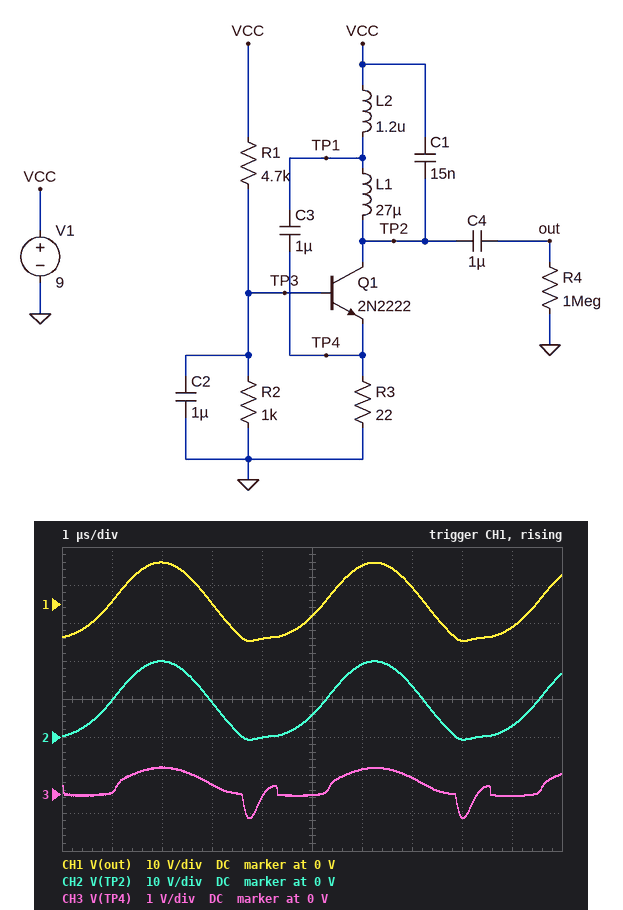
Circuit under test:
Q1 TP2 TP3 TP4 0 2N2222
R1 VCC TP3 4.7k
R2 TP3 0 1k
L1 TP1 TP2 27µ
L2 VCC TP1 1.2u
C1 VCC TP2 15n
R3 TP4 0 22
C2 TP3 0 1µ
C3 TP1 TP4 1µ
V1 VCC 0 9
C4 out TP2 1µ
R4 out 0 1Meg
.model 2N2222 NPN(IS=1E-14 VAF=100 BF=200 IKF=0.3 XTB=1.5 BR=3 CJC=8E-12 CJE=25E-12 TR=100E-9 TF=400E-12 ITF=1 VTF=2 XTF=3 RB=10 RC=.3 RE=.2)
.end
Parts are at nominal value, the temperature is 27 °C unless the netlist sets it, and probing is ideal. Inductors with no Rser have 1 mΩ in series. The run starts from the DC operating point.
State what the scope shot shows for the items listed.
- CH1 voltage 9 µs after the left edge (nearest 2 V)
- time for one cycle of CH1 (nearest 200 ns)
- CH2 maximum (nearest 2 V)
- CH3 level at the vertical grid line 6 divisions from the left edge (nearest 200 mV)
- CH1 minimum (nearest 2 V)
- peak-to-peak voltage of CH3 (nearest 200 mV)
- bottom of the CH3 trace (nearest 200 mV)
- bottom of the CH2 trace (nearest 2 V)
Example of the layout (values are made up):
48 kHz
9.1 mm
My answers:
-6 V
4.2 µs
20 V
600 mV
-10 V
1.4 V
-600 mV
0 V
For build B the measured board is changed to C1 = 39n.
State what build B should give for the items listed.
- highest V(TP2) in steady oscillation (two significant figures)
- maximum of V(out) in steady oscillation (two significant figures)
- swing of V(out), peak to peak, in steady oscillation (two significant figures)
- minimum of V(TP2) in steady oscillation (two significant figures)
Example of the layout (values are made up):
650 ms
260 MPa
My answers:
19 V
10 V
20 V
-720 mV
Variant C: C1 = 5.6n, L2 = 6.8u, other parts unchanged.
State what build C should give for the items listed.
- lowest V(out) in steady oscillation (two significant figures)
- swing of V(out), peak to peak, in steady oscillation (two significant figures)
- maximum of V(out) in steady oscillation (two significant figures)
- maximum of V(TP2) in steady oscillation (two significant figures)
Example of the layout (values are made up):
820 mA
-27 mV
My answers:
-9.9 V
24 V
14 V
23 V
